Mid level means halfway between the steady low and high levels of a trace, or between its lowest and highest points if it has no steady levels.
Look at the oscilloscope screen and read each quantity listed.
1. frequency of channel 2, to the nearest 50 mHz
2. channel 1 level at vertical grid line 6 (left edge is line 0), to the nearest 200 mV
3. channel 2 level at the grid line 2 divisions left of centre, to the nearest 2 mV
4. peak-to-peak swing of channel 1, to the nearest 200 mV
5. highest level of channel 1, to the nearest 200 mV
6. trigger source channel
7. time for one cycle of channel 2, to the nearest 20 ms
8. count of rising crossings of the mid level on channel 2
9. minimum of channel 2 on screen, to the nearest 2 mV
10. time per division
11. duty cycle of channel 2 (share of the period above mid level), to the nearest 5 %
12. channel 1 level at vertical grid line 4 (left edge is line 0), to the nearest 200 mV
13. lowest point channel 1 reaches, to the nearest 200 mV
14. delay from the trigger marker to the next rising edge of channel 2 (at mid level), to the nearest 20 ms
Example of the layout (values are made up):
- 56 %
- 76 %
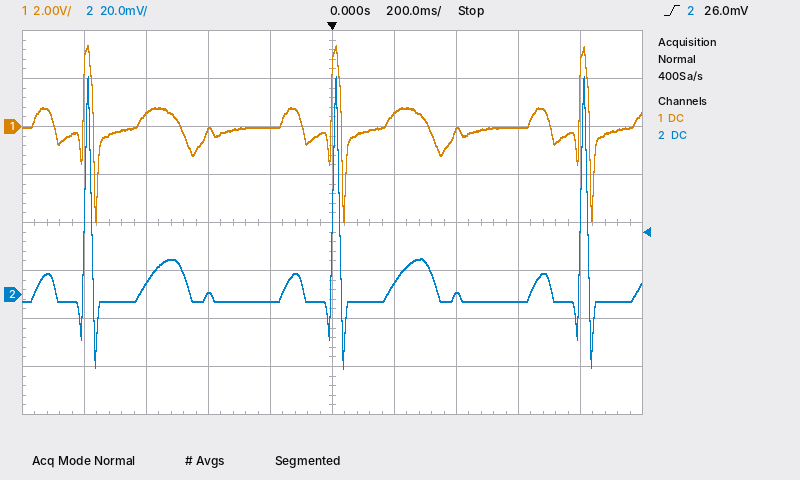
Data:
- 1.25 Hz
- 600 mV
- 0 mV
- 7.4 V
- 3.4 V
- channel 2
- 800 ms
- 3
- -30 mV
- 200 ms
- 5 %
- 0.0 V
- -4.0 V
- 800 ms
